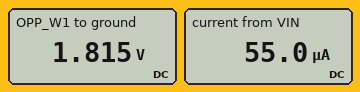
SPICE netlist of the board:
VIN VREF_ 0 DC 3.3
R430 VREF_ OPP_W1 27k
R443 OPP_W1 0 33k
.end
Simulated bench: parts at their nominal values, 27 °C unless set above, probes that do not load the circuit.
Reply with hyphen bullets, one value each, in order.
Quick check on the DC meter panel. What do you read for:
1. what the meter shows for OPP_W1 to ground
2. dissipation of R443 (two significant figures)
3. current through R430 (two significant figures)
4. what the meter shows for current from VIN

- 1.815 V
- 100 µW
- 55 µA
- 55.0 µA
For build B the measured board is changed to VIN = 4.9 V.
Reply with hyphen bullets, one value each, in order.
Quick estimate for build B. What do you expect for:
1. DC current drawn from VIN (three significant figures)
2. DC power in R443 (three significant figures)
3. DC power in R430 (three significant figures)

- 81.7 µA
- 220 µW
- 180 µW
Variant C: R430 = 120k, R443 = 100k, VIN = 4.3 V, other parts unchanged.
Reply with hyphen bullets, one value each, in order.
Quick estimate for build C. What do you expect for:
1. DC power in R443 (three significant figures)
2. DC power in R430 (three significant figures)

- 38.2 µW
- 45.8 µW
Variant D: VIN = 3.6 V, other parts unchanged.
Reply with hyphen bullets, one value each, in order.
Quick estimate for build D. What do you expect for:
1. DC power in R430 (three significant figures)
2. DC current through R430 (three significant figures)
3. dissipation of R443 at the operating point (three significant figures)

- 97.2 µW
- 60.0 µA
- 119 µW
